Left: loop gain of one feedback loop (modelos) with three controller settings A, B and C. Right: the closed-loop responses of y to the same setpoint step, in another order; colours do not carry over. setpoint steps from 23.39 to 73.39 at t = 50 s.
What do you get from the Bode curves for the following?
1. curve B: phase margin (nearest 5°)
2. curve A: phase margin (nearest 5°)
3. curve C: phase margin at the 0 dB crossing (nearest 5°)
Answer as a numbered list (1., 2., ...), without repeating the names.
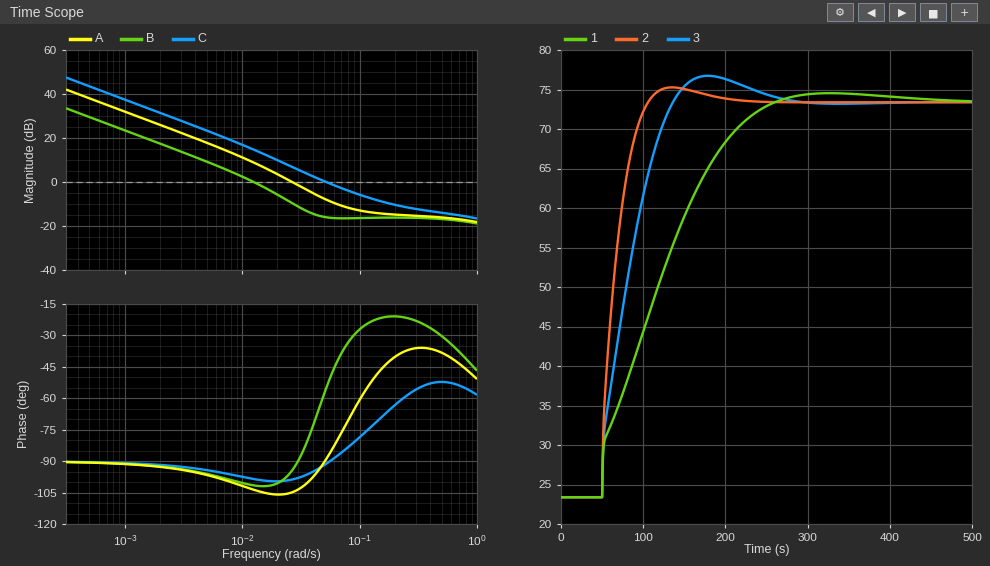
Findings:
1. 80°
2. 75°
3. 90°
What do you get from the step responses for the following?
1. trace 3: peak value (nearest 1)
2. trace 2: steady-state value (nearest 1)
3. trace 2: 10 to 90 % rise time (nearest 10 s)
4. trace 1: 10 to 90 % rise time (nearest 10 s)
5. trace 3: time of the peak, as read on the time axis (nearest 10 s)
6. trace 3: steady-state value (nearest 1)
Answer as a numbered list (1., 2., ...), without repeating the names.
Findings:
1. 77
2. 73
3. 40 s
4. 150 s
5. 180 s
6. 73
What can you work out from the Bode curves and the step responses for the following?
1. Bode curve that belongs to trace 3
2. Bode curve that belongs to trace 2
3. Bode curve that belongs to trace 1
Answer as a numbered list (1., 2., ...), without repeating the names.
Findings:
1. A
2. C
3. B
